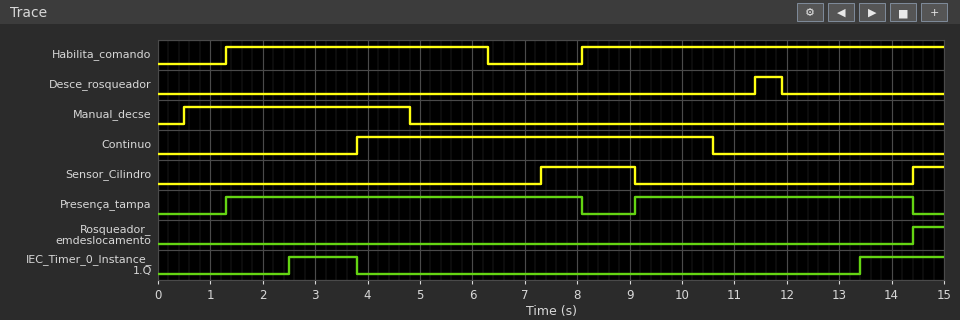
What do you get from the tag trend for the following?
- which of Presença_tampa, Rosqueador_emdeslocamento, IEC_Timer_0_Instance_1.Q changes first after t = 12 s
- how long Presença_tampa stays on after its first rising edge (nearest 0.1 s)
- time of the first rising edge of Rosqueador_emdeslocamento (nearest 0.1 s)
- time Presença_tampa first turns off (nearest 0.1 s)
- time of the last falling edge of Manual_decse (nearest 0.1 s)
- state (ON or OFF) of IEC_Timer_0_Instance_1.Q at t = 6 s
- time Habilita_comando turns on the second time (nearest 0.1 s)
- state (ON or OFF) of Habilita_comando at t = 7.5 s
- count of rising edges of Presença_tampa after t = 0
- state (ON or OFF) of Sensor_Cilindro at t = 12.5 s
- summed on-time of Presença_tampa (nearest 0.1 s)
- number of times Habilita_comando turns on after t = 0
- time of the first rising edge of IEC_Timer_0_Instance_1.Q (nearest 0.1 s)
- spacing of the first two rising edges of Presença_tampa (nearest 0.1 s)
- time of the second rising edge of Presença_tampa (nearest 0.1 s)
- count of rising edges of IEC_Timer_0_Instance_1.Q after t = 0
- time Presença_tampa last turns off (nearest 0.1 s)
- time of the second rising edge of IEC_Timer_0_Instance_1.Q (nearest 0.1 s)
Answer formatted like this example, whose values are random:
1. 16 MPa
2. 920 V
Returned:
1. IEC_Timer_0_Instance_1.Q
2. 6.8 s
3. 14.4 s
4. 8.1 s
5. 4.8 s
6. OFF
7. 8.1 s
8. OFF
9. 2
10. OFF
11. 12.1 s
12. 2
13. 2.5 s
14. 7.8 s
15. 9.1 s
16. 2
17. 14.4 s
18. 13.4 s
